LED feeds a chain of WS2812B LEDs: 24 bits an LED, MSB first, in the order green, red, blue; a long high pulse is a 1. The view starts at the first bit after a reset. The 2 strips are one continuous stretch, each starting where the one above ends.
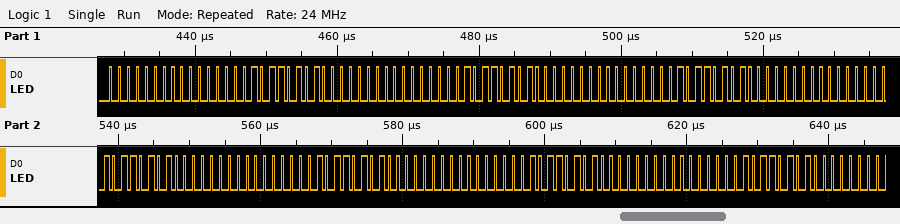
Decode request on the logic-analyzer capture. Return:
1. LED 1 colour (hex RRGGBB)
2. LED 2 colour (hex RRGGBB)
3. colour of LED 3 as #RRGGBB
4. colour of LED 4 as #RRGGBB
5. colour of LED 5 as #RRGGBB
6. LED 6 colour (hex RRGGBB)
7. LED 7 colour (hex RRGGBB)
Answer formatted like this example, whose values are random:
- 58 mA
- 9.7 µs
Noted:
- #0000B5
- #0000B5
- #0000B5
- #0000B5
- #0000B5
- #0000B5
- #0000B5
